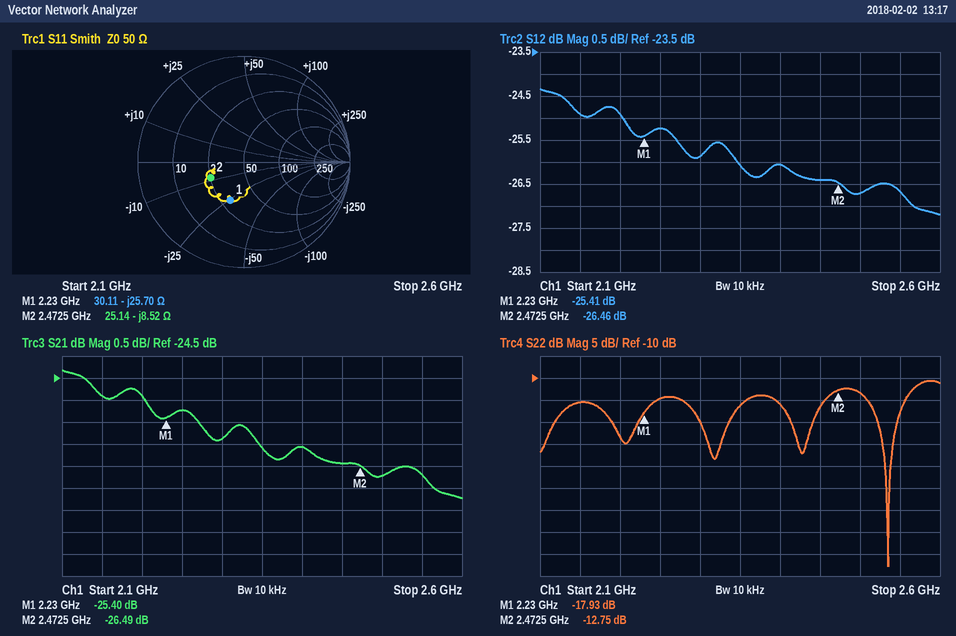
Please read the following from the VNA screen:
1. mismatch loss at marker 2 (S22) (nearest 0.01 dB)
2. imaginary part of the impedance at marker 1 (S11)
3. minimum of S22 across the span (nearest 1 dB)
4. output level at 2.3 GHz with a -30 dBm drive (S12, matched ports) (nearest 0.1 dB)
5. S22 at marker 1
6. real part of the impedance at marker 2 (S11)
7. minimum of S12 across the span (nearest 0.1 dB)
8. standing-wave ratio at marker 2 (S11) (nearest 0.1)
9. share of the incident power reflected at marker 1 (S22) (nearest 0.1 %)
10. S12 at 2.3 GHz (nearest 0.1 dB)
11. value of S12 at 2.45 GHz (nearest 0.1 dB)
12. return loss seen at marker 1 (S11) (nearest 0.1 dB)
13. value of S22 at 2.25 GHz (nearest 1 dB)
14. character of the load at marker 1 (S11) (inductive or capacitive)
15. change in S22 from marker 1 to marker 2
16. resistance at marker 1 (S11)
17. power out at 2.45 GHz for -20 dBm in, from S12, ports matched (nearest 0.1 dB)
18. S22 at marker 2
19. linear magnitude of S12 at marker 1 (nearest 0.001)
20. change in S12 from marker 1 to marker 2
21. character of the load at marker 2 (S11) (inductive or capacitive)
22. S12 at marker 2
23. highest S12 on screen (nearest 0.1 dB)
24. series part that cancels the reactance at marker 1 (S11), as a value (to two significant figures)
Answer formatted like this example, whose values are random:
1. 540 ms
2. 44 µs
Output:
1. 0.24 dB
2. -25.70 Ω
3. -53 dB
4. -55.9 dBm
5. -17.93 dB
6. 25.14 Ω
7. -27.2 dB
8. 2.1
9. 1.6 %
10. -25.9 dB
11. -26.4 dB
12. 8.3 dB
13. -15 dB
14. capacitive
15. 5.18 dB
16. 30.11 Ω
17. -46.4 dBm
18. -12.75 dB
19. 0.054
20. -1.05 dB
21. capacitive
22. -26.46 dB
23. -24.3 dB
24. 1.8 nH
